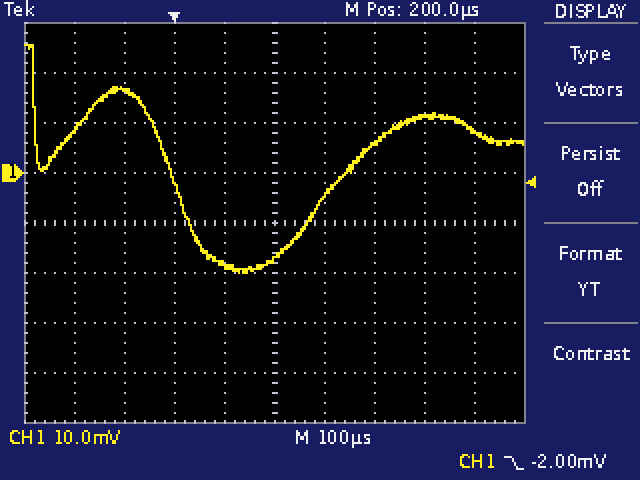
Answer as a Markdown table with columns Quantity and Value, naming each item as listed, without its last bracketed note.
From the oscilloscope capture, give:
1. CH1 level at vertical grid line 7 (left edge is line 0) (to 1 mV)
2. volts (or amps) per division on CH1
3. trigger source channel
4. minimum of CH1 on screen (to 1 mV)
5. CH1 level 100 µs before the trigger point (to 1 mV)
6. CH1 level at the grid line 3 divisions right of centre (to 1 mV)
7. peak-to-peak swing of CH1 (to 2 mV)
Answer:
| Quantity | Value |
|---|---|
| CH1 level at vertical grid line 7 (left edge is line 0) | 6 mV |
| volts (or amps) per division on CH1 | 10 mV |
| trigger source channel | CH1 |
| minimum of CH1 on screen | -20 mV |
| CH1 level 100 µs before the trigger point | 17 mV |
| CH1 level at the grid line 3 divisions right of centre | 11 mV |
| peak-to-peak swing of CH1 | 46 mV |
